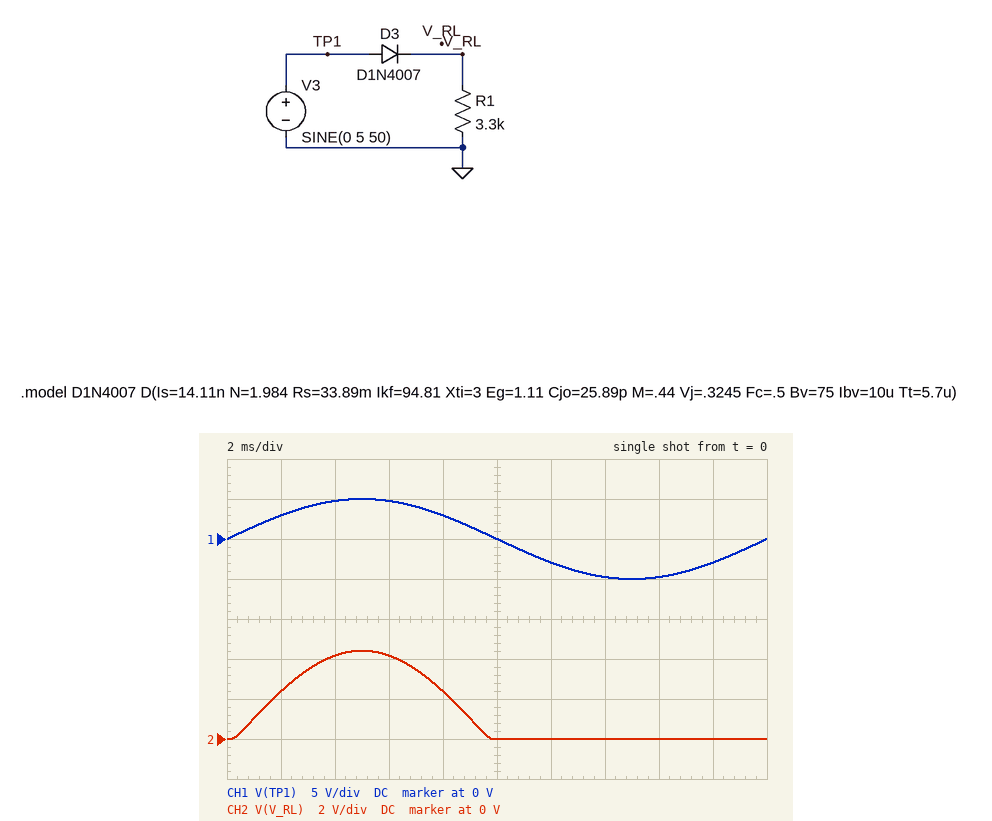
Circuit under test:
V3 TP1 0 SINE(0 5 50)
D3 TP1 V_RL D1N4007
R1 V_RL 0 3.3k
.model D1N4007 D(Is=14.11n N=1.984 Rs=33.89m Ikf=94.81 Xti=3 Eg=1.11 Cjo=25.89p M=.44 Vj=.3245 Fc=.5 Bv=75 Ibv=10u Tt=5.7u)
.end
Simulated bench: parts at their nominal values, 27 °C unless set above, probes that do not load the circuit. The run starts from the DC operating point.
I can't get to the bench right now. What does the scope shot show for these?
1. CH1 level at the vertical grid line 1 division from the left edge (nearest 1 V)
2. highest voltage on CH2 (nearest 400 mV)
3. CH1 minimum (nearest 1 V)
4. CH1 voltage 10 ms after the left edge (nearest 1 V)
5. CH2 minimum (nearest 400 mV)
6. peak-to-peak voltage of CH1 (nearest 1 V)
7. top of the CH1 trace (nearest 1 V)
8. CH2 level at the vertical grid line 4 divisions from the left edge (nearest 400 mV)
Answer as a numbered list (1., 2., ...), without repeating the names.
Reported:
1. 3 V
2. 4.4 V
3. -5 V
4. 0 V
5. 0 V
6. 10 V
7. 5 V
8. 2.4 V
